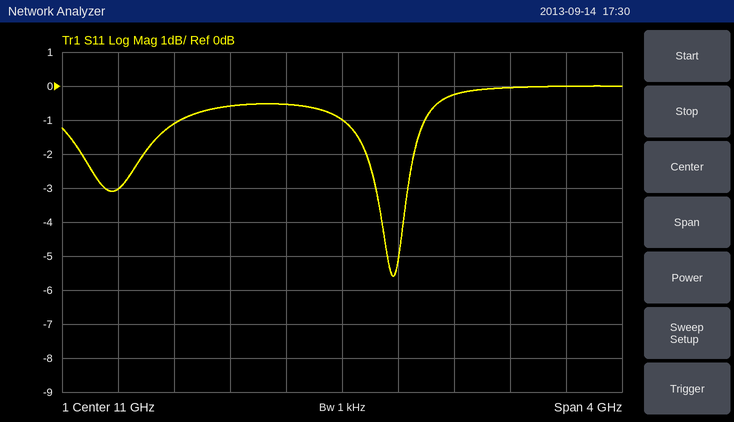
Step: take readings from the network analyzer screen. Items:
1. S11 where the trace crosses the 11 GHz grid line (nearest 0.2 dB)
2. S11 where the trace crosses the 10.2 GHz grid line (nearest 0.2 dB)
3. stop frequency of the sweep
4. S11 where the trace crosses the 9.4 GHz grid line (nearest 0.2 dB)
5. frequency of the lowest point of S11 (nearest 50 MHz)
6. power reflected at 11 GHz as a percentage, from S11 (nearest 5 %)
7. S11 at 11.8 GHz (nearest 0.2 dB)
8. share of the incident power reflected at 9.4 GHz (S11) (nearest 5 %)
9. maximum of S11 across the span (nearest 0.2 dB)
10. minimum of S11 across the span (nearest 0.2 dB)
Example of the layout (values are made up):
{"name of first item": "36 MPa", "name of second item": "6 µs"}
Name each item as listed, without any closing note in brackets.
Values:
{"S11 where the trace crosses the 11 GHz grid line": "-1.0 dB", "S11 where the trace crosses the 10.2 GHz grid line": "-0.6 dB", "stop frequency of the sweep": "13 GHz", "S11 where the trace crosses the 9.4 GHz grid line": "-3.0 dB", "frequency of the lowest point of S11": "11.35 GHz", "power reflected at 11 GHz as a percentage, from S11": "80 %", "S11 at 11.8 GHz": "-0.2 dB", "share of the incident power reflected at 9.4 GHz (S11)": "50 %", "maximum of S11 across the span": "0.0 dB", "minimum of S11 across the span": "-5.6 dB"}
